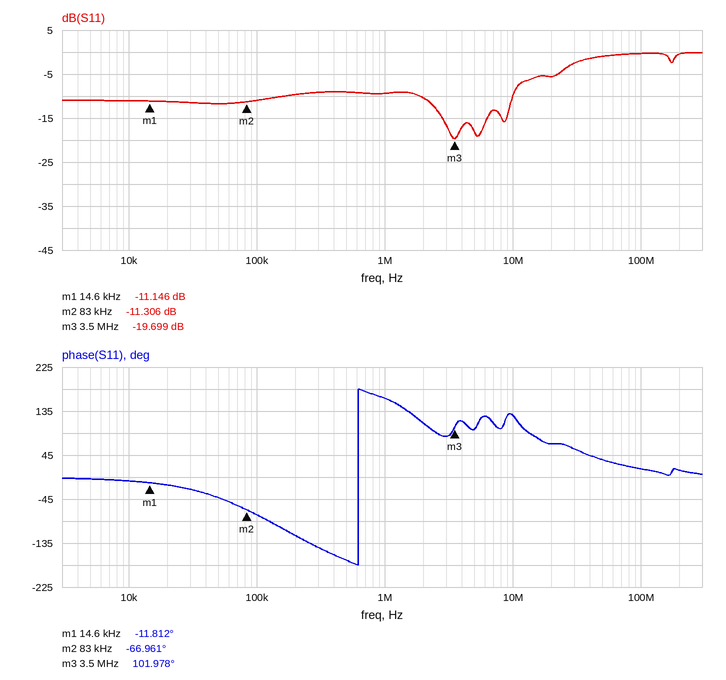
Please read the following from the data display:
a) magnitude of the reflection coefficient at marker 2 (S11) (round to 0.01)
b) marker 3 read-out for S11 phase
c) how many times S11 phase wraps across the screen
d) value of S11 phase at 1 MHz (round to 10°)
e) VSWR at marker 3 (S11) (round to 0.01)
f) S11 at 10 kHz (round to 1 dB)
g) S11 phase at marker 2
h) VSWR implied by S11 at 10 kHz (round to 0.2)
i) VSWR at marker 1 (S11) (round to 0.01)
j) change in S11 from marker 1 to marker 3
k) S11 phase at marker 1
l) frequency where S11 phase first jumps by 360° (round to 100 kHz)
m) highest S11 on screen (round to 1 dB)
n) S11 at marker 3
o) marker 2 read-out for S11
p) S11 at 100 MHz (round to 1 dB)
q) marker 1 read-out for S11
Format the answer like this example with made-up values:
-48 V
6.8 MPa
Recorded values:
0.27
101.978°
1
160°
1.23
-11 dB
-66.961°
1.8
1.77
-8.553 dB
-11.812°
600 kHz
0 dB
-19.699 dB
-11.306 dB
0 dB
-11.146 dB
